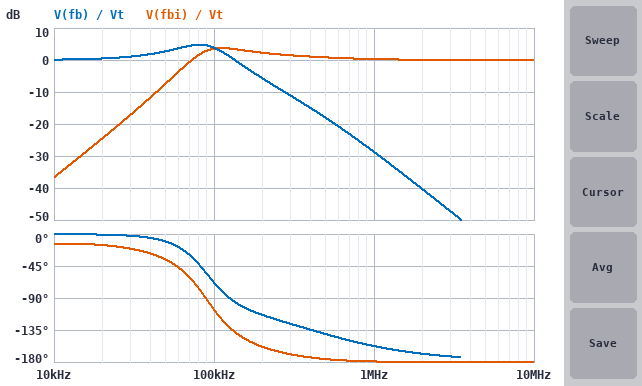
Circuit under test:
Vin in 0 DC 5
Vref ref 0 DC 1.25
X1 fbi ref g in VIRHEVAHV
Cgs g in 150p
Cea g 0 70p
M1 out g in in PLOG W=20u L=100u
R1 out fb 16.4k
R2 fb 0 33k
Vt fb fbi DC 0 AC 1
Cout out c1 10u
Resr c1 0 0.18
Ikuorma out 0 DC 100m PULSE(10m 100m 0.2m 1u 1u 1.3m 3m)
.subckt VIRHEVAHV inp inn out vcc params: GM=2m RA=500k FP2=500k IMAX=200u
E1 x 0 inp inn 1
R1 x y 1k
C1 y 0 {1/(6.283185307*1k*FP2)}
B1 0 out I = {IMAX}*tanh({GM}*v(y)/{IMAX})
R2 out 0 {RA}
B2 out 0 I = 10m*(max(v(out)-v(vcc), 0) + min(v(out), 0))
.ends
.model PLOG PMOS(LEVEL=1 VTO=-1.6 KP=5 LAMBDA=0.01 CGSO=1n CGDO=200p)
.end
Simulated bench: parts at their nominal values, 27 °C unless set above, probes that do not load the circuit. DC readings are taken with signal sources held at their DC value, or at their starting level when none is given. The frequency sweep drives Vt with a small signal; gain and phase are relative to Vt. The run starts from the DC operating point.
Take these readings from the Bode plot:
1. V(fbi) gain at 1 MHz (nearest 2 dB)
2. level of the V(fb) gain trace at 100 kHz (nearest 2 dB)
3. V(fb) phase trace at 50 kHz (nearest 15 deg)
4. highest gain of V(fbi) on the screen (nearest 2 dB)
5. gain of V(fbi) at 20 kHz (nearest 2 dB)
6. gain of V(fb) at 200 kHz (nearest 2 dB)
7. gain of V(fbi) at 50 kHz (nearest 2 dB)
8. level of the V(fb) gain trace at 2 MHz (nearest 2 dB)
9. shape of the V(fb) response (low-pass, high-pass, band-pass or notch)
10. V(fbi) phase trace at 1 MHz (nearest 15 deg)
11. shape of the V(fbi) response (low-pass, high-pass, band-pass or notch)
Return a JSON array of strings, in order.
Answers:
["0 dB", "4 dB", "-15 deg", "4 dB", "-24 dB", "-6 dB", "-8 dB", "-40 dB", "low-pass", "-180 deg", "high-pass"]
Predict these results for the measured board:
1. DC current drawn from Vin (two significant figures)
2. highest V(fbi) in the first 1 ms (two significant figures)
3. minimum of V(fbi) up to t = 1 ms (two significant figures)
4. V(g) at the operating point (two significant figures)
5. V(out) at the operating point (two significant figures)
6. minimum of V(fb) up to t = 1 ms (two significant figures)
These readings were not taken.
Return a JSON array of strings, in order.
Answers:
["100 mA", "1.3 V", "1.2 V", "3.0 V", "1.9 V", "1.2 V"]
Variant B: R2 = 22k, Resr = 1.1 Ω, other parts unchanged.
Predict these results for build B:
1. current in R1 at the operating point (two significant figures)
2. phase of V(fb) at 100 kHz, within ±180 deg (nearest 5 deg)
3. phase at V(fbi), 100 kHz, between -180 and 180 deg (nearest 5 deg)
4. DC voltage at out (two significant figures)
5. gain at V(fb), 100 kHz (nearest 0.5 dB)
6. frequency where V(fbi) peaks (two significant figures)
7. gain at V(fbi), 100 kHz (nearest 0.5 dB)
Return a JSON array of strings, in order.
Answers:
["57 µA", "-15 deg", "-85 deg", "2.2 V", "0.5 dB", "530 kHz", "-12.0 dB"]
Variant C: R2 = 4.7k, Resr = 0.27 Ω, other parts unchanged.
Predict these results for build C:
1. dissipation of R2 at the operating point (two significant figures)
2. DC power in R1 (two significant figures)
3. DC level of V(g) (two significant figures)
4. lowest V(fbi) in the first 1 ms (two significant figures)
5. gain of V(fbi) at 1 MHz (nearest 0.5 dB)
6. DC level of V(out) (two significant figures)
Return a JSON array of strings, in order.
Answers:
["260 µW", "910 µW", "-18 mV", "1.1 V", "0 dB", "5.0 V"]
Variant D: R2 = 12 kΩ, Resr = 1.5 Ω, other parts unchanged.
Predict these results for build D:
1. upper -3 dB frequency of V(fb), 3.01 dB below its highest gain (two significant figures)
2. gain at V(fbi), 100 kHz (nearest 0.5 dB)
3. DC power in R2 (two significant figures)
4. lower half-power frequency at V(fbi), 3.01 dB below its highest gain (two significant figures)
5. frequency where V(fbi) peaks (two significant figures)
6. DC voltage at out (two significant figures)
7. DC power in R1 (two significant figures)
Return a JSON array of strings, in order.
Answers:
["520 kHz", "-12.0 dB", "130 µW", "320 kHz", "530 kHz", "3.0 V", "180 µW"]
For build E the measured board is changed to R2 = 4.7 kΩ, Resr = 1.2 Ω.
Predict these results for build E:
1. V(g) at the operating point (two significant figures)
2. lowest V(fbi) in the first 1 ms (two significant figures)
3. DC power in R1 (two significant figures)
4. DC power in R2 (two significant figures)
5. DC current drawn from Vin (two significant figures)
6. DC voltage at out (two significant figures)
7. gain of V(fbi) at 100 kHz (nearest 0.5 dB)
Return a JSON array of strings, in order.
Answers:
["-18 mV", "1.1 V", "910 µW", "260 µW", "100 mA", "5.0 V", "0 dB"]
